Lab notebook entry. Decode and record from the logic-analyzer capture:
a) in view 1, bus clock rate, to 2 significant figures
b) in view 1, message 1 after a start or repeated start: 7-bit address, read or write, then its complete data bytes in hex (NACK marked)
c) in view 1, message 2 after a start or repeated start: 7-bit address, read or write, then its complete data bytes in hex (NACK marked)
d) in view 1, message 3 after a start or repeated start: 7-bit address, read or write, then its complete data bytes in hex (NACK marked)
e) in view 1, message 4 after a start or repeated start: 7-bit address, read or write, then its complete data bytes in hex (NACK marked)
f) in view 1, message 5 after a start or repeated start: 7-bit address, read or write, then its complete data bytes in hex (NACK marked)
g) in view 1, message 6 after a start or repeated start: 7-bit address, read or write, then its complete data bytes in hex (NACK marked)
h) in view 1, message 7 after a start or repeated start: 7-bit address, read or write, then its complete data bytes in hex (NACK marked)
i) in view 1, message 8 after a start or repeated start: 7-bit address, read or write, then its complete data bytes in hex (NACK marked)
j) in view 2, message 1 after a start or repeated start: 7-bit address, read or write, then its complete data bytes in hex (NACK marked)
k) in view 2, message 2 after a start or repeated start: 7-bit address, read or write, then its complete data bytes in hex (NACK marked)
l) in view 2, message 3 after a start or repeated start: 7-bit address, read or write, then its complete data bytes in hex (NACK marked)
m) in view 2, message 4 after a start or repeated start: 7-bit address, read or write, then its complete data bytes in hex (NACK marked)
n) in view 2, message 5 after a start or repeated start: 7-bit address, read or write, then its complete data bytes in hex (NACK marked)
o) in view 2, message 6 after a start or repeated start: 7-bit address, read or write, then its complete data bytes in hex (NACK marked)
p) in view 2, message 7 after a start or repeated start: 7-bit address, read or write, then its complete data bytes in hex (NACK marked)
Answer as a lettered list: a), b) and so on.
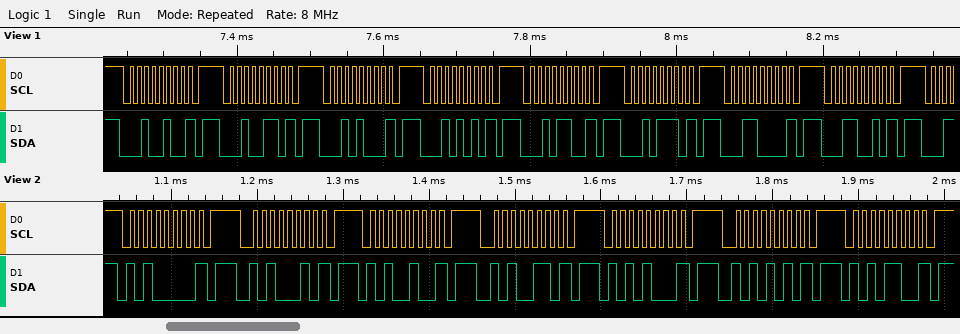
a) 100 kHz
b) 0x12 write NACK
c) 0x13 write NACK
d) 0x14 write NACK
e) 0x15 write NACK
f) 0x16 write NACK
g) 0x17 write NACK
h) 0x18 write NACK
i) 0x19 write NACK
j) 0x50 write NACK
k) 0x51 write NACK
l) 0x52 write NACK
m) 0x53 write NACK
n) 0x54 write NACK
o) 0x55 write NACK
p) 0x56 write NACK
